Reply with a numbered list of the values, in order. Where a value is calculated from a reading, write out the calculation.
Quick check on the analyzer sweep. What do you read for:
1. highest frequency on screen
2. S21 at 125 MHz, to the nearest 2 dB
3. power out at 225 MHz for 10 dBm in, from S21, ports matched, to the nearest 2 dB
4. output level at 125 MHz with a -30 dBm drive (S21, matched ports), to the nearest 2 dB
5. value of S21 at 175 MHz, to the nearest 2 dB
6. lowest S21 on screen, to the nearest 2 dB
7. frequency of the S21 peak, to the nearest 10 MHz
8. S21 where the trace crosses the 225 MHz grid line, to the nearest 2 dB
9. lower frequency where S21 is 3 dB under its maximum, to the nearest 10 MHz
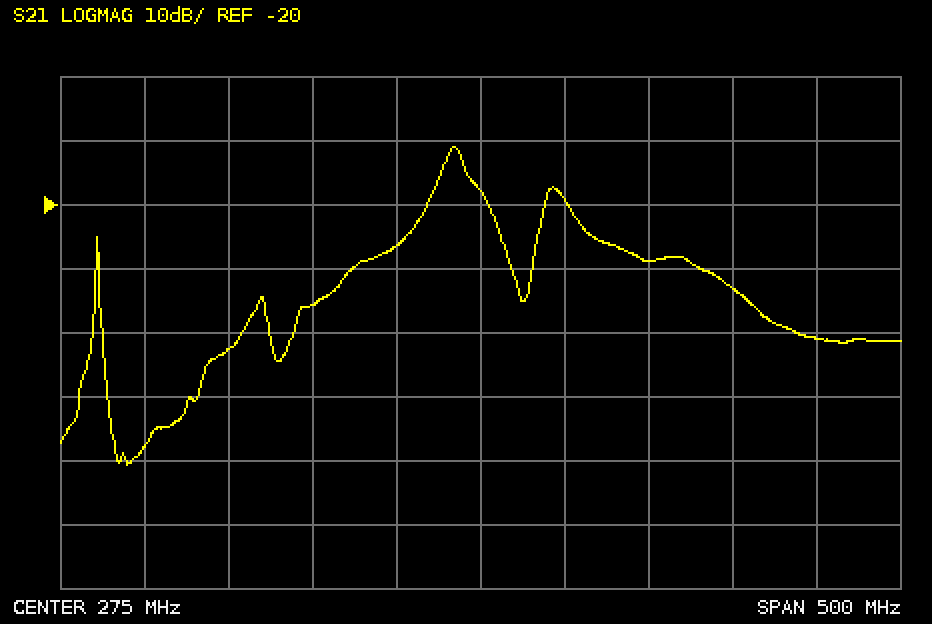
1. 525 MHz
2. -42 dB
3. 10 dBm + (-26 dB) = -16 dBm
4. -30 dBm + (-42 dB) = -72 dBm
5. -36 dB
6. -60 dB
7. 260 MHz
8. -26 dB
9. 250 MHz
